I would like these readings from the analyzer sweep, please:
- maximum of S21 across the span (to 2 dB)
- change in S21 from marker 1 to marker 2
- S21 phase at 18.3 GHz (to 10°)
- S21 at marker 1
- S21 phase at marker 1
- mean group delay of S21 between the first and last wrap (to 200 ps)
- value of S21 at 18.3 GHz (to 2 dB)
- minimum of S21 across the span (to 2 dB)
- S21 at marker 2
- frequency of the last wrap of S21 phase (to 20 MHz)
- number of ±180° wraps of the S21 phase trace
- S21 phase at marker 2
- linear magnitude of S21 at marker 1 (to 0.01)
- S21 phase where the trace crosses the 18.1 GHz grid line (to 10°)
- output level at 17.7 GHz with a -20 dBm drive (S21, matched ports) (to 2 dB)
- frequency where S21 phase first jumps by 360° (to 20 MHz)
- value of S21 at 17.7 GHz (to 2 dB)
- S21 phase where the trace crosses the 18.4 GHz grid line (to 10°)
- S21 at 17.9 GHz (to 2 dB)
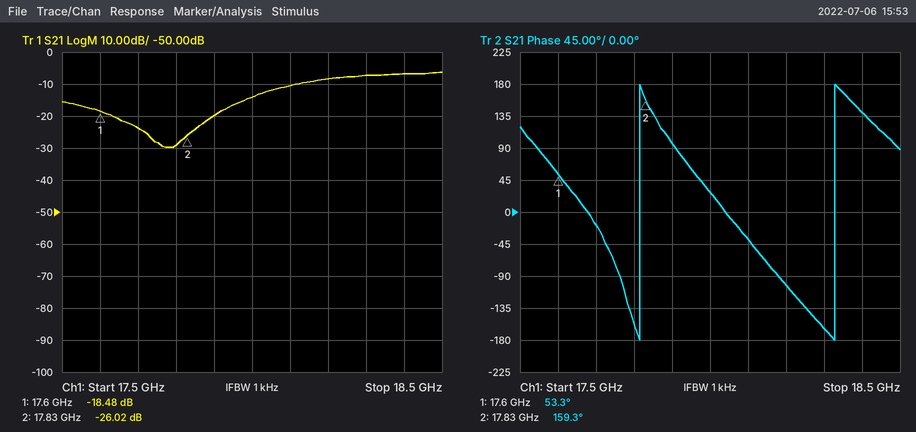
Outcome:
-6 dB
-7.54 dB
-160°
-18.48 dB
53.3°
2.0 ns
-8 dB
-30 dB
-26.02 dB
18.32 GHz
2
159.3°
0.12
-40°
-44 dBm
17.82 GHz
-24 dB
140°
-20 dB
